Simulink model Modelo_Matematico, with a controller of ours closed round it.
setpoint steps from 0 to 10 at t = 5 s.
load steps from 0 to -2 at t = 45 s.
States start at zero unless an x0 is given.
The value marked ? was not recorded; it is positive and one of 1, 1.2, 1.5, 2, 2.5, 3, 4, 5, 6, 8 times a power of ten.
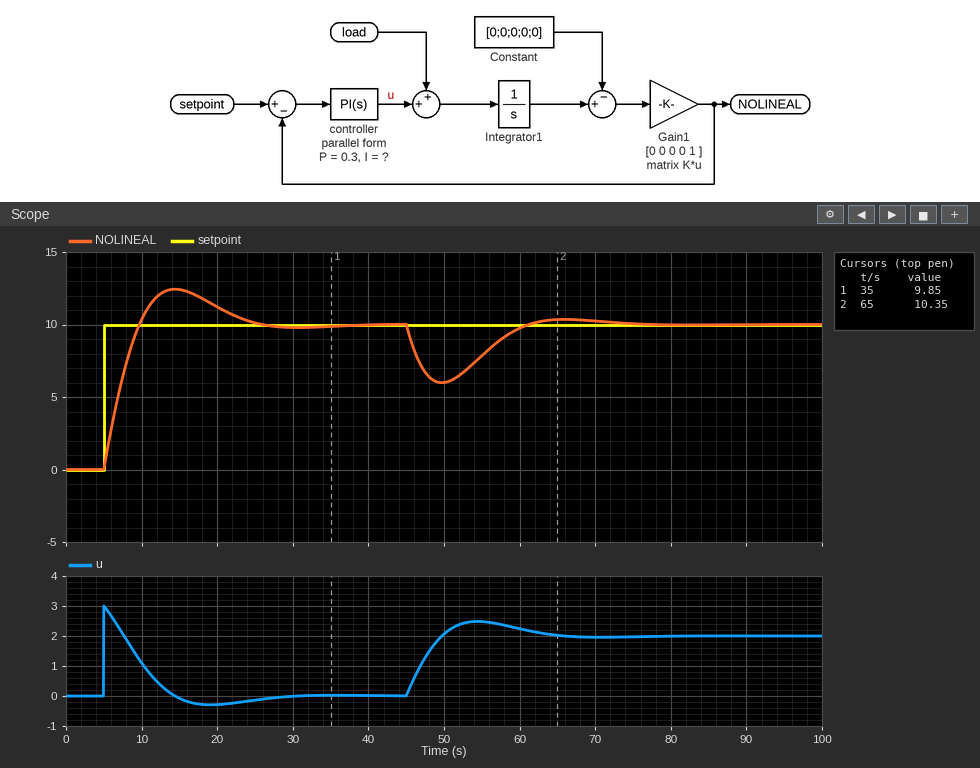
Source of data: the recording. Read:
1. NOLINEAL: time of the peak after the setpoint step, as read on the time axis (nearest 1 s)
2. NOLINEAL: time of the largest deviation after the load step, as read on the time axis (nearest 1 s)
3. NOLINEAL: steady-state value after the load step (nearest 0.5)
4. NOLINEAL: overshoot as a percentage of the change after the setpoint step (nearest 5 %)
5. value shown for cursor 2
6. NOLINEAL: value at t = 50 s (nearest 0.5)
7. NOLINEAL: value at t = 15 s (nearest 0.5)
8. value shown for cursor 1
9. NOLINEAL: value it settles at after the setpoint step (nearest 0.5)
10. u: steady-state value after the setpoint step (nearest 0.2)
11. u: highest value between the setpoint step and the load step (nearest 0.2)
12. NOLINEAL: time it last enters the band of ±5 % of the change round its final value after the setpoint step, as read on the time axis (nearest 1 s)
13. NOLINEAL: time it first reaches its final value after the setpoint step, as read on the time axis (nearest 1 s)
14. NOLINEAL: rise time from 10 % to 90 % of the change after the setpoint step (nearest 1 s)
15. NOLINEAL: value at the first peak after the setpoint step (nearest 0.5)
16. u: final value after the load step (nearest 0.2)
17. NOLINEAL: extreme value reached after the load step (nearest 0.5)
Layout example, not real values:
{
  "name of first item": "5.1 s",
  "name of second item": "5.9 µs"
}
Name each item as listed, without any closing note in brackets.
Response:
{
  "NOLINEAL: time of the peak after the setpoint step, as read on the time axis": "14 s",
  "NOLINEAL: time of the largest deviation after the load step, as read on the time axis": "50 s",
  "NOLINEAL: steady-state value after the load step": "10.0",
  "NOLINEAL: overshoot as a percentage of the change after the setpoint step": "25 %",
  "value shown for cursor 2": "10.35",
  "NOLINEAL: value at t = 50 s": "6.0",
  "NOLINEAL: value at t = 15 s": "12.5",
  "value shown for cursor 1": "9.85",
  "NOLINEAL: value it settles at after the setpoint step": "10.0",
  "u: steady-state value after the setpoint step": "0.0",
  "u: highest value between the setpoint step and the load step": "3.0",
  "NOLINEAL: time it last enters the band of ±5 % of the change round its final value after the setpoint step, as read on the time axis": "23 s",
  "NOLINEAL: time it first reaches its final value after the setpoint step, as read on the time axis": "10 s",
  "NOLINEAL: rise time from 10 % to 90 % of the change after the setpoint step": "4 s",
  "NOLINEAL: value at the first peak after the setpoint step": "12.5",
  "u: final value after the load step": "2.0",
  "NOLINEAL: extreme value reached after the load step": "6.0"
}
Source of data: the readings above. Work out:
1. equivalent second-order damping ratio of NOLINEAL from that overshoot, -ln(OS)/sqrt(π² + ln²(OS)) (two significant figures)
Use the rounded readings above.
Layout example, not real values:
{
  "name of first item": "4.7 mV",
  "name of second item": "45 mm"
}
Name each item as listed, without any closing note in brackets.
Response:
{
  "equivalent second-order damping ratio of NOLINEAL from that overshoot, -ln(OS)/sqrt(π² + ln²(OS))": "0.40"
}
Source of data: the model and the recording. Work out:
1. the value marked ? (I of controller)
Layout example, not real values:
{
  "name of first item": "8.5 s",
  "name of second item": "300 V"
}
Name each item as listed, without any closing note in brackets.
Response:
{
  "the value marked ?": "0.06"
}
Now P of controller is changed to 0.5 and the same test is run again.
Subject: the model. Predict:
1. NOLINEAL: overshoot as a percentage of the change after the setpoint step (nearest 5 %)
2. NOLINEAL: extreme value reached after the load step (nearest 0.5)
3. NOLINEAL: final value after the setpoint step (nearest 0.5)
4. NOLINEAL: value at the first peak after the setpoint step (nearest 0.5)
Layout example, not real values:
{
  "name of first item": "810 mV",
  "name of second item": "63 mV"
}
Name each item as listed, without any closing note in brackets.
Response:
{
  "NOLINEAL: overshoot as a percentage of the change after the setpoint step": "15 %",
  "NOLINEAL: extreme value reached after the load step": "7.0",
  "NOLINEAL: final value after the setpoint step": "10.0",
  "NOLINEAL: value at the first peak after the setpoint step": "11.5"
}
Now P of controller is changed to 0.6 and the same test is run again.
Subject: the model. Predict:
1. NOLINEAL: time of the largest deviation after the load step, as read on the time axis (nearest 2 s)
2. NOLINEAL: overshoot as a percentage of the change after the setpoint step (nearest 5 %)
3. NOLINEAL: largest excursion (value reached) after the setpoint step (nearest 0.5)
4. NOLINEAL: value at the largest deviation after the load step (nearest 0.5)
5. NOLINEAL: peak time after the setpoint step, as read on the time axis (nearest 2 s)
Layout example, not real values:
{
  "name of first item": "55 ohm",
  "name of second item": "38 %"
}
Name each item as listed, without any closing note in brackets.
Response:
{
  "NOLINEAL: time of the largest deviation after the load step, as read on the time axis": "48 s",
  "NOLINEAL: overshoot as a percentage of the change after the setpoint step": "10 %",
  "NOLINEAL: largest excursion (value reached) after the setpoint step": "11.0",
  "NOLINEAL: value at the largest deviation after the load step": "7.5",
  "NOLINEAL: peak time after the setpoint step, as read on the time axis": "12 s"
}
